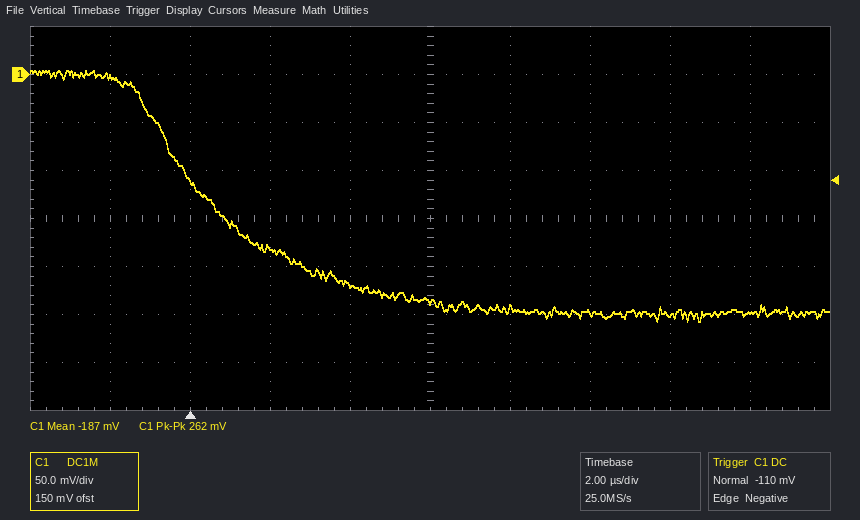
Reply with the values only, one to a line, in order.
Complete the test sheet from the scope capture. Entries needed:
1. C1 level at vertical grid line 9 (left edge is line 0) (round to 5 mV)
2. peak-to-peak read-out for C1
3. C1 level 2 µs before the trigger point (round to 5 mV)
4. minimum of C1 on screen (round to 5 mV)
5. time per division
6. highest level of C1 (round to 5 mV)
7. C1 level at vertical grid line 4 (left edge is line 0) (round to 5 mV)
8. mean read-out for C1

-250 mV
262 mV
0 mV
-255 mV
2 µs
5 mV
-220 mV
-187 mV
